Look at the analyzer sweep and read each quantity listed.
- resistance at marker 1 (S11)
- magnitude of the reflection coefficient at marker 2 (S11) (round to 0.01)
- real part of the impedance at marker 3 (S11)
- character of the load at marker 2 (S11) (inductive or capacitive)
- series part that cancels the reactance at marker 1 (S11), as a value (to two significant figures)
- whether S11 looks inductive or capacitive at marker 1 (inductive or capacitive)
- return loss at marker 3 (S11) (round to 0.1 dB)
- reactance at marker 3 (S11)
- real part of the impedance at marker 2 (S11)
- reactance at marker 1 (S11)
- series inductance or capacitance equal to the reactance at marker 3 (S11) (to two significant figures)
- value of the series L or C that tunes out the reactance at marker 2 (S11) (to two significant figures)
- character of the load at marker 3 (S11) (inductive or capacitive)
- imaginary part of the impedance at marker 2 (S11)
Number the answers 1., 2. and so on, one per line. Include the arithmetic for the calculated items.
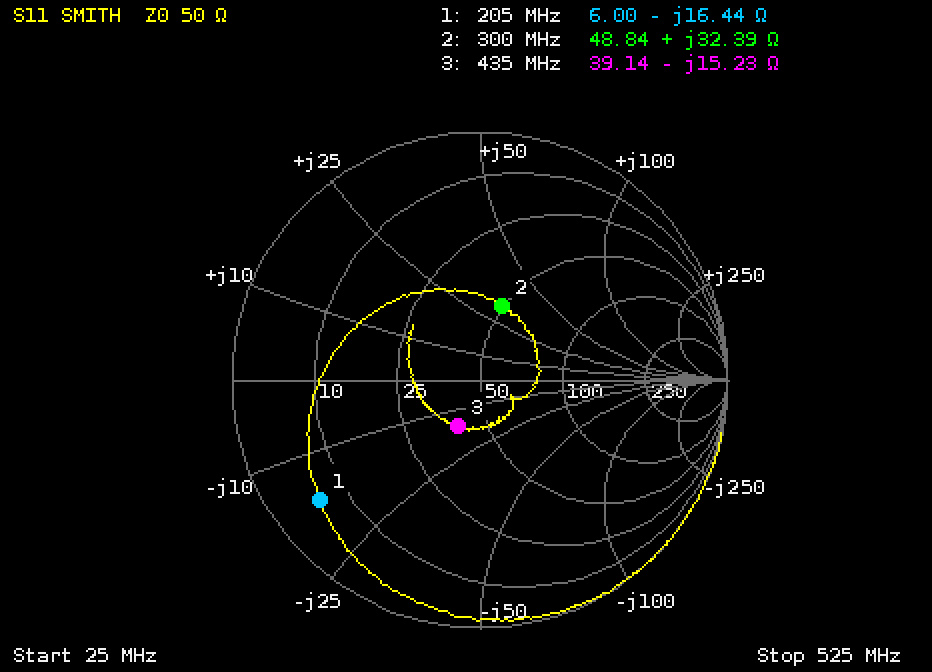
1. 6.00 Ω
2. 0.31
3. 39.14 Ω
4. inductive
5. L = 16.44 Ω/(2π × 205 MHz) ≈ 13 nH
6. capacitive
7. 13.7 dB
8. -15.23 Ω
9. 48.84 Ω
10. -16.44 Ω
11. C = 1/(2π × 435 MHz × 15.23 Ω) ≈ 24 pF
12. C = 1/(2π × 300 MHz × 32.39 Ω) ≈ 16 pF
13. capacitive
14. +32.39 Ω
